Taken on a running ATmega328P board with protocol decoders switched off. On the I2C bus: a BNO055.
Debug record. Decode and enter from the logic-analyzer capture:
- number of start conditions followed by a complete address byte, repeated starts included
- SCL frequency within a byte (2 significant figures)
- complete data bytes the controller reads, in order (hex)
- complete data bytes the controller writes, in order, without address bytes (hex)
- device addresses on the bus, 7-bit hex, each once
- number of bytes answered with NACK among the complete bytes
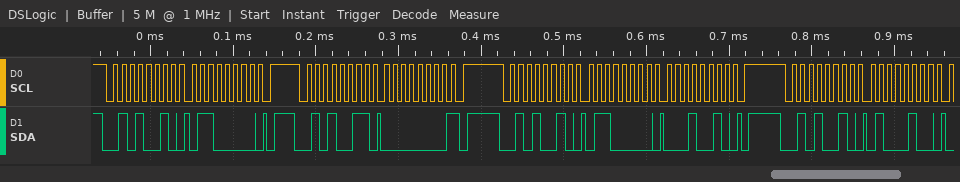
4
100 kHz
00
60 60 12 44
0x29
1
